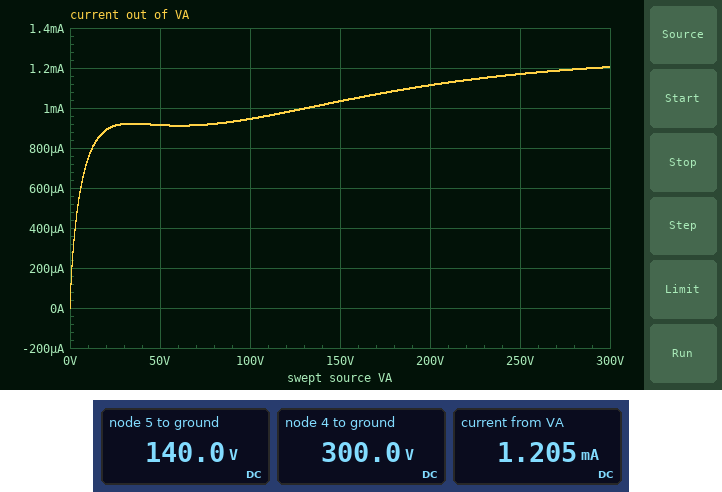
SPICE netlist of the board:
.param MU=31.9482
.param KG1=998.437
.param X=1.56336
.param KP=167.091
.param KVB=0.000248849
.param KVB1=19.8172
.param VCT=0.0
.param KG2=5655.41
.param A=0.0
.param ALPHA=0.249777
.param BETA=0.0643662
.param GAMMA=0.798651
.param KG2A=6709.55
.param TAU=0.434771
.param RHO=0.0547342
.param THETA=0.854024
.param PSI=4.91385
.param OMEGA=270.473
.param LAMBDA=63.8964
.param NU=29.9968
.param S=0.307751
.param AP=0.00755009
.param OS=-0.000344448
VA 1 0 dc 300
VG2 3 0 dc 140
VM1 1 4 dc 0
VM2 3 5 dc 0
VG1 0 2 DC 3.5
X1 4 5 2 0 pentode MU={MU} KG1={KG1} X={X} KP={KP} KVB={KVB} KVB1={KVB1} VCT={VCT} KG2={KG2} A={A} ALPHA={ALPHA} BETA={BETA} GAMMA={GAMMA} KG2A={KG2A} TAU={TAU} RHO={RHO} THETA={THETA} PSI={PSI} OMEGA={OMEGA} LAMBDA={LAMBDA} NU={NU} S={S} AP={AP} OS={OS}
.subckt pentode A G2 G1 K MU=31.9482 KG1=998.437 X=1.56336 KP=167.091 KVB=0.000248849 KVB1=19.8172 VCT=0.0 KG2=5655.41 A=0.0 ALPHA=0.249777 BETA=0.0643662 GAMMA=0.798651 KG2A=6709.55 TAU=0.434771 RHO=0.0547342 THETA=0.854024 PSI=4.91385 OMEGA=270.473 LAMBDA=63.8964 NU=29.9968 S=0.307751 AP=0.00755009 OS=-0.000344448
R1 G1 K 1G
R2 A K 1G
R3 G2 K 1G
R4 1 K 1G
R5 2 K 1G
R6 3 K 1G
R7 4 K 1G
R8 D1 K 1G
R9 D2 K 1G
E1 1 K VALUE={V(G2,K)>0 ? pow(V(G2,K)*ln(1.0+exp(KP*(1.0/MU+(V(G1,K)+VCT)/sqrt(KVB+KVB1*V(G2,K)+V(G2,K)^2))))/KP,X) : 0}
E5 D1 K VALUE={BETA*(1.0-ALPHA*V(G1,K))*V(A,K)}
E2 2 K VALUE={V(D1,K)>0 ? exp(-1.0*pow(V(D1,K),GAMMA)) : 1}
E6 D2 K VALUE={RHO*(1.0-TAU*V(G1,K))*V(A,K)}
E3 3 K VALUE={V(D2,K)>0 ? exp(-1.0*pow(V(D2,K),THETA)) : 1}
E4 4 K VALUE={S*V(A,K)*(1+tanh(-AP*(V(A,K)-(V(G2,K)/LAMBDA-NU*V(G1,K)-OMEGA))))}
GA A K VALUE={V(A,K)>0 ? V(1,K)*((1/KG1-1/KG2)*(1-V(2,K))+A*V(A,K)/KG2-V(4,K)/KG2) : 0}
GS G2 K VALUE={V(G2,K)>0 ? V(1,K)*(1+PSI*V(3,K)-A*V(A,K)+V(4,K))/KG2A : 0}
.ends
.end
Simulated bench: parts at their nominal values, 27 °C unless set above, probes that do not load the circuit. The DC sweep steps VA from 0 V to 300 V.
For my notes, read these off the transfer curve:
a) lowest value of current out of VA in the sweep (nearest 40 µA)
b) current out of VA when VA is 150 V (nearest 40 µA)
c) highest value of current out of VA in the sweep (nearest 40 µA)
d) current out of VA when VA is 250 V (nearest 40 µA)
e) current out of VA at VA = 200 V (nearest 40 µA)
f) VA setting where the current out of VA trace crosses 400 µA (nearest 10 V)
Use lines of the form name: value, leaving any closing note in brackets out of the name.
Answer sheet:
lowest value of current out of VA in the sweep: 0 A
current out of VA when VA is 150 V: 1.04 mA
highest value of current out of VA in the sweep: 1.20 mA
current out of VA when VA is 250 V: 1.16 mA
current out of VA at VA = 200 V: 1.12 mA
VA setting where the current out of VA trace crosses 400 µA: 0 V
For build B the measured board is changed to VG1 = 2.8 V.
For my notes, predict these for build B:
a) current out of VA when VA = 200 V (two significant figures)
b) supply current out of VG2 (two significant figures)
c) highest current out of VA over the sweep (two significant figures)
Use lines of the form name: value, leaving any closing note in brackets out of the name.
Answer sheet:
current out of VA when VA = 200 V: 2.0 mA
supply current out of VG2: 440 µA
highest current out of VA over the sweep: 2.1 mA
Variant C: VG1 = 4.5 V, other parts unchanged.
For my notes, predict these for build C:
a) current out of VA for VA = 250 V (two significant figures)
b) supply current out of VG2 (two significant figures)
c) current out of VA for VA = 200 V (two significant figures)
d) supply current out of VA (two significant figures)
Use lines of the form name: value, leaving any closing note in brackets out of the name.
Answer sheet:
current out of VA for VA = 250 V: 400 µA
supply current out of VG2: 100 µA
current out of VA for VA = 200 V: 370 µA
supply current out of VA: 420 µA
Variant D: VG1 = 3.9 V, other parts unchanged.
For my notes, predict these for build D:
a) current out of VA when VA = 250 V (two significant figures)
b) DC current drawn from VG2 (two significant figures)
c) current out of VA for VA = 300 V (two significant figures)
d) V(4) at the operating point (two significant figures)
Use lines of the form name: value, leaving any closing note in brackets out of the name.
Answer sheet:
current out of VA when VA = 250 V: 790 µA
DC current drawn from VG2: 190 µA
current out of VA for VA = 300 V: 820 µA
V(4) at the operating point: 300 V
